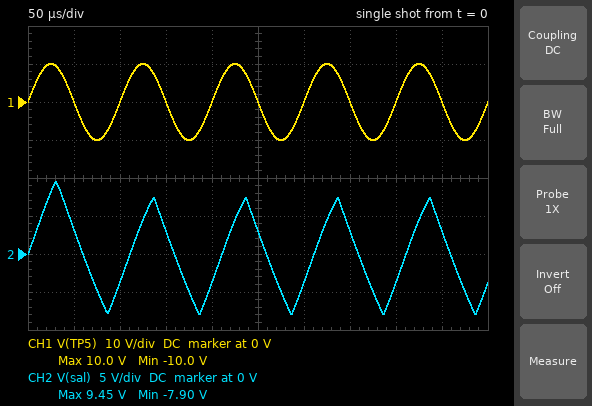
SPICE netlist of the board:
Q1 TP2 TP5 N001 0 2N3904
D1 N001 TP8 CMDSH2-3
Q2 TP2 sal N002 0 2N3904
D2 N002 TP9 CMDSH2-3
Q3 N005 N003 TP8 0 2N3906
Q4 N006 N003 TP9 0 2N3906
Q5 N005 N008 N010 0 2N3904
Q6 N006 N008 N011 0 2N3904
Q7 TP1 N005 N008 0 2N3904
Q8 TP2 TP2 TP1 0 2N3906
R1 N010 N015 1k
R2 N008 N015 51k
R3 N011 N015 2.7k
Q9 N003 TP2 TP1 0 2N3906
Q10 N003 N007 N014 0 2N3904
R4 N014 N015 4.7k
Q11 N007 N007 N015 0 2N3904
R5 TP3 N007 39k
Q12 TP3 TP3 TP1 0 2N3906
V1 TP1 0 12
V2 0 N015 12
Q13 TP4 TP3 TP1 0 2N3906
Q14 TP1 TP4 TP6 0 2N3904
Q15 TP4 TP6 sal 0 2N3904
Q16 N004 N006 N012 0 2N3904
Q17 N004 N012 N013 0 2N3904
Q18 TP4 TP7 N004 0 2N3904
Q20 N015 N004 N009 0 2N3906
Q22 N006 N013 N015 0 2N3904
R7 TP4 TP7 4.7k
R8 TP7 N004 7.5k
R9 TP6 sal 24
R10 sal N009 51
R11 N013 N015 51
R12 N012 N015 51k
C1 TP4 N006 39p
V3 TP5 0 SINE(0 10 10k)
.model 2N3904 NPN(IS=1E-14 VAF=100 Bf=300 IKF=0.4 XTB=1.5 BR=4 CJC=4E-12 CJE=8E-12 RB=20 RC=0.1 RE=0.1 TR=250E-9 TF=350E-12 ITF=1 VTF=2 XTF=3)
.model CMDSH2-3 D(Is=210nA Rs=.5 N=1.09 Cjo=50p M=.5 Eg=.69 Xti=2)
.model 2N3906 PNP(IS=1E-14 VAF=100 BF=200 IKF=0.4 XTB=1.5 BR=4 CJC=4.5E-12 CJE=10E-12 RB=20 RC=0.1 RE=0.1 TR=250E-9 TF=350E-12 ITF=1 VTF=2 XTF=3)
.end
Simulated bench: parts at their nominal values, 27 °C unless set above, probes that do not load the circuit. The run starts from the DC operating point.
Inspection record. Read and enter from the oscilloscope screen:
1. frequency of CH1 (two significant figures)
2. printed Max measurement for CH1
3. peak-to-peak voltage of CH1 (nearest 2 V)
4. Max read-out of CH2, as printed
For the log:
10 kHz
10.0 V
20 V
9.45 V
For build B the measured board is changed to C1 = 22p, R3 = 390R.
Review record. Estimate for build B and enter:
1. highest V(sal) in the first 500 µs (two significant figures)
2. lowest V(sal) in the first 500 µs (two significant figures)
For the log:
10 V
-10 V
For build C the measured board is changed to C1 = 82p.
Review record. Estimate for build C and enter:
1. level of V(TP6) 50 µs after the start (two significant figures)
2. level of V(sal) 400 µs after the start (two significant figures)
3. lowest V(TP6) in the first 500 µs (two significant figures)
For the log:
3.9 V
-4.1 V
-5.5 V
